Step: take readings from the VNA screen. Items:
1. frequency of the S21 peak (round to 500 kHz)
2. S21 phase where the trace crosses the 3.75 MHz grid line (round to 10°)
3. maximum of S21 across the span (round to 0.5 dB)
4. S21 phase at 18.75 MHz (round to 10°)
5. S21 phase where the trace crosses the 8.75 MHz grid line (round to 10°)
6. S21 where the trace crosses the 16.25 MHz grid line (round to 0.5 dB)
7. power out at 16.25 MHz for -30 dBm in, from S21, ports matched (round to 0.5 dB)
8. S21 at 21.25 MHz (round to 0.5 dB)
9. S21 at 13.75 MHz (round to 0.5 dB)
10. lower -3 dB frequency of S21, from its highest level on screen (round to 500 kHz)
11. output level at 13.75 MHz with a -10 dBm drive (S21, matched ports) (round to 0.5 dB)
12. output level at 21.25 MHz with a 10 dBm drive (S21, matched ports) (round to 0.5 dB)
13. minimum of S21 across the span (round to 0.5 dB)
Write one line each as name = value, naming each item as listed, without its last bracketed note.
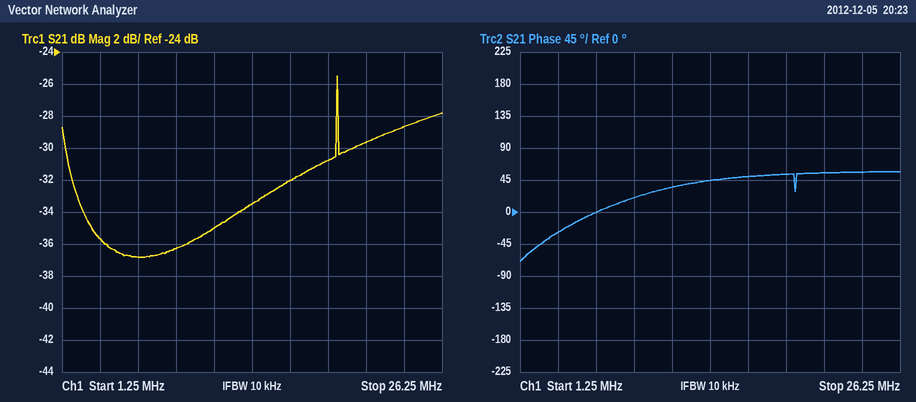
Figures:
frequency of the S21 peak = 19.5 MHz
S21 phase where the trace crosses the 3.75 MHz grid line = -30°
maximum of S21 across the span = -25.5 dB
S21 phase at 18.75 MHz = 50°
S21 phase where the trace crosses the 8.75 MHz grid line = 20°
S21 where the trace crosses the 16.25 MHz grid line = -32.0 dB
power out at 16.25 MHz for -30 dBm in, from S21, ports matched = -62.0 dBm
S21 at 21.25 MHz = -29.5 dB
S21 at 13.75 MHz = -33.5 dB
lower -3 dB frequency of S21, from its highest level on screen = 19.5 MHz
output level at 13.75 MHz with a -10 dBm drive (S21, matched ports) = -43.5 dBm
output level at 21.25 MHz with a 10 dBm drive (S21, matched ports) = -19.5 dBm
minimum of S21 across the span = -37.0 dB
